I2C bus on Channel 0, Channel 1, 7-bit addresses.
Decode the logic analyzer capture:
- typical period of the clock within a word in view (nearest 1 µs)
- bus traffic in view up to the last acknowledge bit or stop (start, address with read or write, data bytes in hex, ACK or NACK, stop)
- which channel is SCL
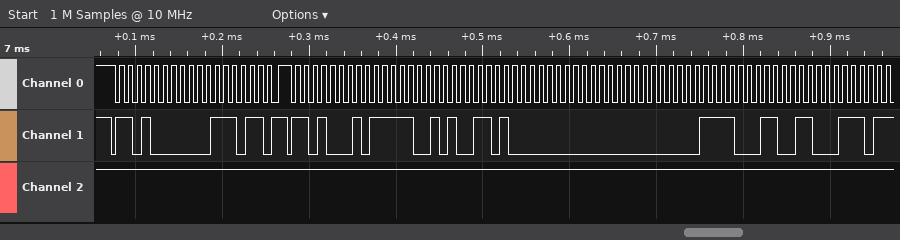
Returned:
10 µs
start, address 68 write ACK, 3B ACK, repeated start, address 68 read ACK, F9 ACK, 9A ACK, 00 ACK, 00 ACK, 3C ACK, CC ACK
Channel 0
